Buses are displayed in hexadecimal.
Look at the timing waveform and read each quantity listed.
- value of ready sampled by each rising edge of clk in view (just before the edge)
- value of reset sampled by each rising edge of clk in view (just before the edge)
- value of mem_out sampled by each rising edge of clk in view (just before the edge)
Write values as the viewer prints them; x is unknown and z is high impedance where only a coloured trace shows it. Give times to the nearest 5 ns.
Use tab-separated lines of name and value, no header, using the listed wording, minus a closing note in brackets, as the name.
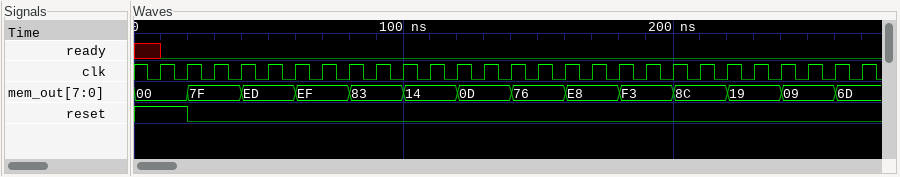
value of ready sampled by each rising edge of clk in view	x 0 0 0 0 0 0 0 0 0 0 0 0 0 0 0 0 0 0 0 0 0 0 0 0 0 0
value of reset sampled by each rising edge of clk in view	1 1 0 0 0 0 0 0 0 0 0 0 0 0 0 0 0 0 0 0 0 0 0 0 0 0 0
value of mem_out sampled by each rising edge of clk in view	00, 00, 7F, 7F, ED, ED, EF, EF, 83, 83, 14, 14, 0D, 0D, 76, 76, E8, E8, F3, F3, 8C, 8C, 19, 19, 09, 09, 6D
